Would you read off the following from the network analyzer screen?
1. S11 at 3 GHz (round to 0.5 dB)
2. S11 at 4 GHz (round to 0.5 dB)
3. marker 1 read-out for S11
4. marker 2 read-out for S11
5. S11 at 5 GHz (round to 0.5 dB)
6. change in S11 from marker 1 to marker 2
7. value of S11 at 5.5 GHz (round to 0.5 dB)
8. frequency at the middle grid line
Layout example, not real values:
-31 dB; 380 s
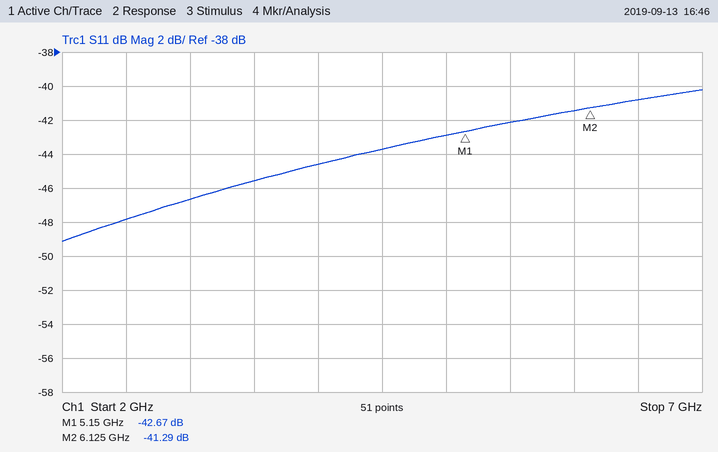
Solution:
-46.5 dB; -44.5 dB; -42.67 dB; -41.29 dB; -43.0 dB; 1.38 dB; -42.0 dB; 4.5 GHz
